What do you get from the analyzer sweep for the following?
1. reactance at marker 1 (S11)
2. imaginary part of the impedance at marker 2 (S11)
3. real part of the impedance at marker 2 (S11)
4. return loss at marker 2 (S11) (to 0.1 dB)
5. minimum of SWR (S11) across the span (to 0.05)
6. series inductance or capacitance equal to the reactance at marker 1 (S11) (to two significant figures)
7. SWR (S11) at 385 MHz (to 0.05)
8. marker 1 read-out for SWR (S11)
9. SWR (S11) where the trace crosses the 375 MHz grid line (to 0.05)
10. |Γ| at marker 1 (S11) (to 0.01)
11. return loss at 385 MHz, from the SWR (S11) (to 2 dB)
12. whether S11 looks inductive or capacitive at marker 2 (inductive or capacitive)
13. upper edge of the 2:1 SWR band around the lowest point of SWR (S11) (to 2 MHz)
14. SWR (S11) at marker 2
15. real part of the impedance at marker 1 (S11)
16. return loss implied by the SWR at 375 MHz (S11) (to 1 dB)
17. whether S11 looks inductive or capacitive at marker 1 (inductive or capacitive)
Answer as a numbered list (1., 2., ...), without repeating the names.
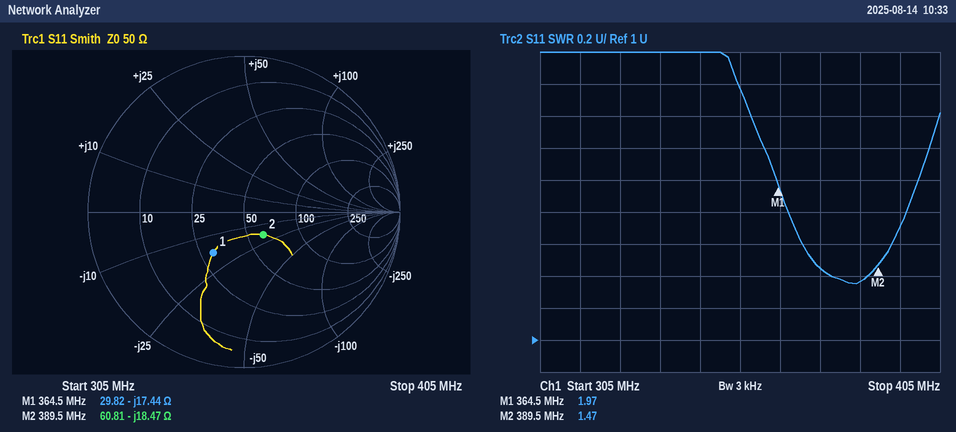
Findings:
1. -17.44 Ω
2. -18.47 Ω
3. 60.81 Ω
4. 14.4 dB
5. 1.35
6. 25 pF
7. 1.35
8. 1.97
9. 1.45
10. 0.33
11. 16 dB
12. capacitive
13. 400 MHz
14. 1.47
15. 29.82 Ω
16. 15 dB
17. capacitive
